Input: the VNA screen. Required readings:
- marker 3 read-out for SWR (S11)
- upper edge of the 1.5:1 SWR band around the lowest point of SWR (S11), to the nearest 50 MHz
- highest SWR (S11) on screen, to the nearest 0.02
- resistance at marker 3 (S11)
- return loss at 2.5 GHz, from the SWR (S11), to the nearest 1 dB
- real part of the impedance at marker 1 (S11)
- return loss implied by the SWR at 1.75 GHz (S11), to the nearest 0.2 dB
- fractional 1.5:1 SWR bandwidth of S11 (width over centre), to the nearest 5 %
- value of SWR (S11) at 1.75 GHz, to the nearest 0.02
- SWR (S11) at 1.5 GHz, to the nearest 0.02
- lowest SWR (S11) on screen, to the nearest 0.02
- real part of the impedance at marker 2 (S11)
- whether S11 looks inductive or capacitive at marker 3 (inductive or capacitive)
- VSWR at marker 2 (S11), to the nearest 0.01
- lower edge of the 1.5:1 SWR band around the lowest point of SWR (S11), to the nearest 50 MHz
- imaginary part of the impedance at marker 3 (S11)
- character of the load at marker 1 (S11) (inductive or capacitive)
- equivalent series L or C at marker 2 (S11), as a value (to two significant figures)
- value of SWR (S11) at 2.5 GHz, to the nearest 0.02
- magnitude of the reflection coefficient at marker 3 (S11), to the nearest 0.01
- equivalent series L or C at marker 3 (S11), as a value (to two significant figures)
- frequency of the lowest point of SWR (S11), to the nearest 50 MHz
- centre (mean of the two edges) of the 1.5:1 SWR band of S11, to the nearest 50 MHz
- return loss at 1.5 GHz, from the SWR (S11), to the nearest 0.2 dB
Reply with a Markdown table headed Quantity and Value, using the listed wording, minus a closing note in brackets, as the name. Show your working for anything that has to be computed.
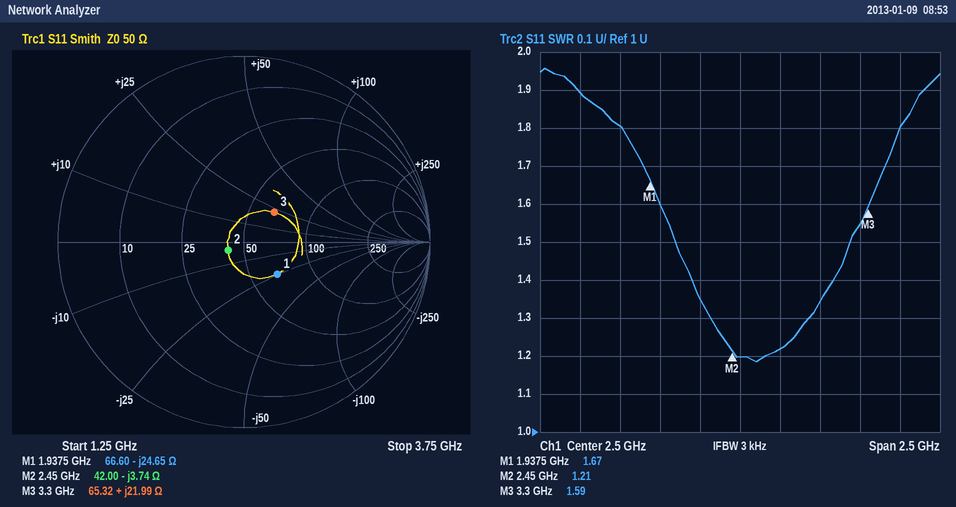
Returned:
| Quantity | Value |
|---|---|
| marker 3 read-out for SWR | 1.59 |
| upper edge of the 1.5:1 SWR band around the lowest point of SWR (S11), to the nearest 50 MHz | 3.20 GHz |
| highest SWR (S11) on screen, to the nearest 0.02 | 1.96 |
| resistance at marker 3 | 65.32 Ω |
| return loss at 2.5 GHz, from the SWR (S11), to the nearest 1 dB | −20 log10((1.2 − 1)/(1.2 + 1)) ≈ 21 dB |
| real part of the impedance at marker 1 | 66.60 Ω |
| return loss implied by the SWR at 1.75 GHz (S11), to the nearest 0.2 dB | −20 log10((1.8 − 1)/(1.8 + 1)) ≈ 10.9 dB, so 10.8 dB to the nearest 0.2 dB |
| fractional 1.5:1 SWR bandwidth of S11 (width over centre), to the nearest 5 % | 1.1 GHz / 2.65 GHz ≈ 41.5 %, so 40 % to the nearest 5 % |
| value of SWR (S11) at 1.75 GHz, to the nearest 0.02 | 1.80 |
| SWR (S11) at 1.5 GHz, to the nearest 0.02 | 1.90 |
| lowest SWR (S11) on screen, to the nearest 0.02 | 1.18 |
| real part of the impedance at marker 2 | 42.00 Ω |
| whether S11 looks inductive or capacitive at marker 3 | inductive |
| VSWR at marker 2 (S11), to the nearest 0.01 | 1.21 |
| lower edge of the 1.5:1 SWR band around the lowest point of SWR (S11), to the nearest 50 MHz | 2.10 GHz |
| imaginary part of the impedance at marker 3 | +21.99 Ω |
| character of the load at marker 1 (S11) | capacitive |
| equivalent series L or C at marker 2 (S11), as a value | C = 1/(2π × 2.45 GHz × 3.74 Ω) ≈ 17 pF |
| value of SWR (S11) at 2.5 GHz, to the nearest 0.02 | 1.20 |
| magnitude of the reflection coefficient at marker 3 (S11), to the nearest 0.01 | 0.23 |
| equivalent series L or C at marker 3 (S11), as a value | L = 21.99 Ω/(2π × 3.3 GHz) ≈ 1.1 nH |
| frequency of the lowest point of SWR (S11), to the nearest 50 MHz | 2.60 GHz |
| centre (mean of the two edges) of the 1.5:1 SWR band of S11, to the nearest 50 MHz | 2.65 GHz |
| return loss at 1.5 GHz, from the SWR (S11), to the nearest 0.2 dB | −20 log10((1.9 − 1)/(1.9 + 1)) ≈ 10.2 dB |
